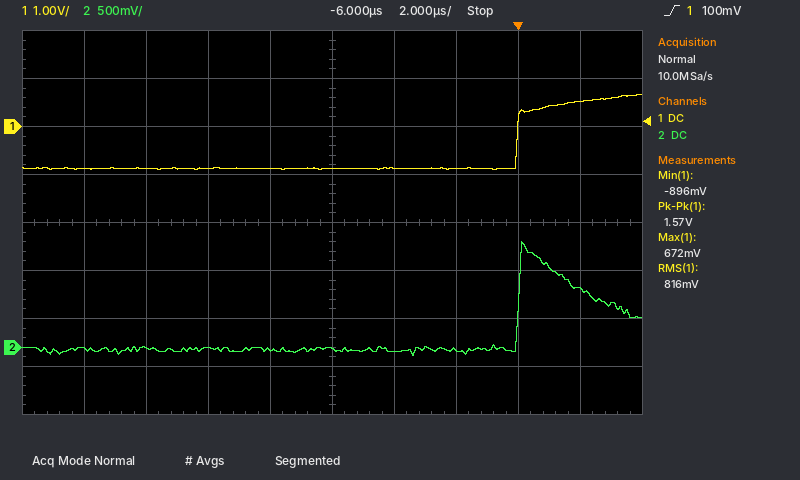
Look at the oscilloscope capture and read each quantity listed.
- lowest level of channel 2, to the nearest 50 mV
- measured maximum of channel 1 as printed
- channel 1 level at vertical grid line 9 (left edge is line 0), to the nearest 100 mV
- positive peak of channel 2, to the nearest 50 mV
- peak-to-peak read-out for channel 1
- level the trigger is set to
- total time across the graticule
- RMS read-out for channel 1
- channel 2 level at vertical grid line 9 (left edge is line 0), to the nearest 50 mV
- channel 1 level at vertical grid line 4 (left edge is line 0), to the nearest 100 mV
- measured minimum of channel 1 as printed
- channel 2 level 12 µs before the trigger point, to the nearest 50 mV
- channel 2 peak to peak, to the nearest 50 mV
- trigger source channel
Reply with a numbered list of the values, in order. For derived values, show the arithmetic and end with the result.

1. -100 mV
2. 672 mV
3. 500 mV
4. 1.10 V
5. 1.57 V
6. 100 mV
7. 20 µs
8. 816 mV
9. 600 mV
10. -900 mV
11. -896 mV
12. 0 mV
13. 1.10 V − (-100 mV) = 1.20 V
14. channel 1
